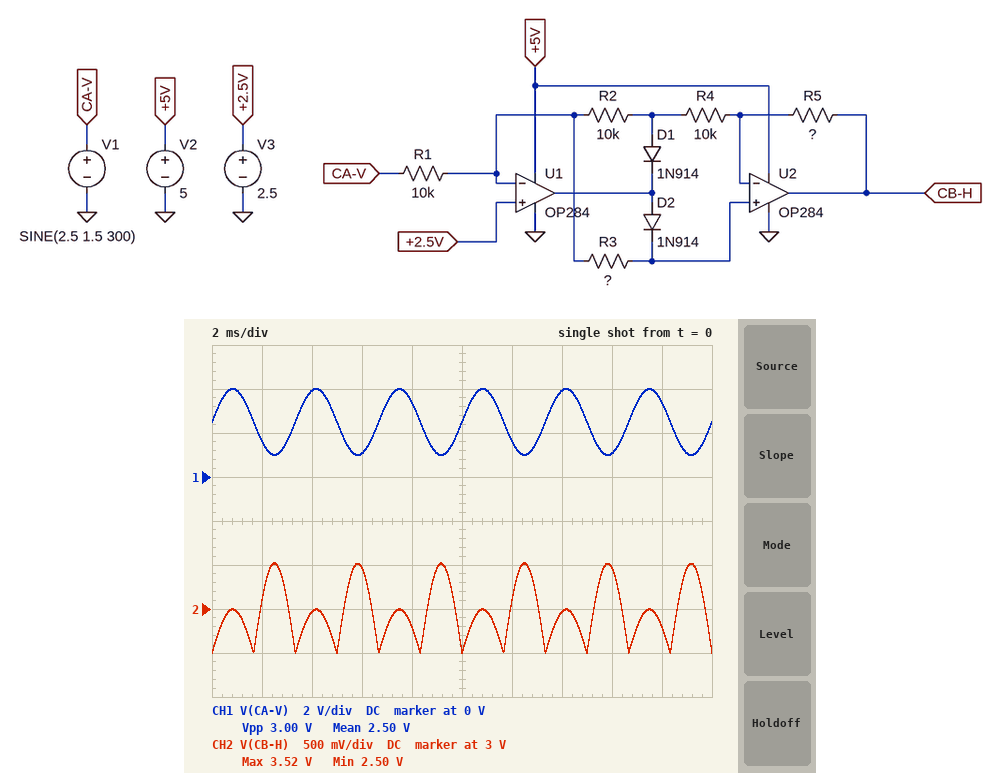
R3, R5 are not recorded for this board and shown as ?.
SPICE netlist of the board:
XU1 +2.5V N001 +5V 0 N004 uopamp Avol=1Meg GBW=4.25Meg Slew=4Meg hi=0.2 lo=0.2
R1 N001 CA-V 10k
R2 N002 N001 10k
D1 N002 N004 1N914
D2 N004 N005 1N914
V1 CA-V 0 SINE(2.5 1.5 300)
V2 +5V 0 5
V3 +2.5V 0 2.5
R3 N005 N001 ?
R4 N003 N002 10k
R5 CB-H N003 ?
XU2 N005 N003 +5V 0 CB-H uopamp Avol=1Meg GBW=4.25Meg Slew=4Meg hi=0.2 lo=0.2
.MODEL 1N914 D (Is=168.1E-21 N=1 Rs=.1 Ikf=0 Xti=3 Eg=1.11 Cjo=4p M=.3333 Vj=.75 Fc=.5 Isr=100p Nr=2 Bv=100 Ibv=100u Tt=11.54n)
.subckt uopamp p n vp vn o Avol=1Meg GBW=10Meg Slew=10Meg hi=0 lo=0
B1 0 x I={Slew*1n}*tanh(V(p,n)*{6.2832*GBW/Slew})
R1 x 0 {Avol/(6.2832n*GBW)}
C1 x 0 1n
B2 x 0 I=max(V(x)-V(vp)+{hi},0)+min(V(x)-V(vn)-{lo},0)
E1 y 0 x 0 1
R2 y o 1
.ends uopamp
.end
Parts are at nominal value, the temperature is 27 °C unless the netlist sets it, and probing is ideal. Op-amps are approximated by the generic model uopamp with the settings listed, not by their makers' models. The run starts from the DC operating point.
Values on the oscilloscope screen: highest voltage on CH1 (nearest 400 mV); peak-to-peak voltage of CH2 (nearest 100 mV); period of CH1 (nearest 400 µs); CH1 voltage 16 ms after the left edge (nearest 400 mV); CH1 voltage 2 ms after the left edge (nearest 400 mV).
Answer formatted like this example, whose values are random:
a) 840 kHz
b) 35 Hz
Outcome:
a) 4.0 V
b) 1.0 V
c) 3.2 ms
d) 1.2 V
e) 1.6 V
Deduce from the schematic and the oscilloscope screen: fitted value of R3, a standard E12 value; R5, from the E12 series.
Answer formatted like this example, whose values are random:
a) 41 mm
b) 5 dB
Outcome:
a) 8.2 kΩ
b) 3.3 kΩ
